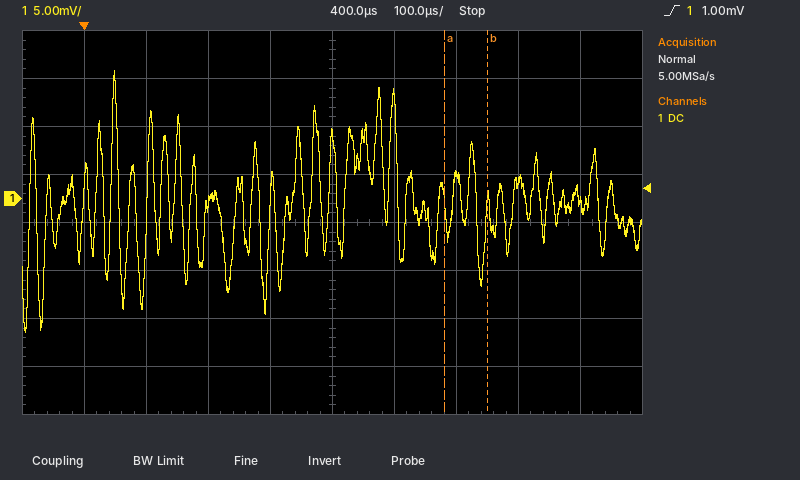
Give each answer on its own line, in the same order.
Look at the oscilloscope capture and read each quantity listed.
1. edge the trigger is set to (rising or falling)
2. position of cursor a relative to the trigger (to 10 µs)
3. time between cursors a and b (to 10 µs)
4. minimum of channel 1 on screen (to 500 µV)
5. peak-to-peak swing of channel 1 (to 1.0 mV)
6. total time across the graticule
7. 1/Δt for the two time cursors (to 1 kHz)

rising
+580 µs
70 µs
-14.0 mV
27.0 mV
1 ms
14 kHz
